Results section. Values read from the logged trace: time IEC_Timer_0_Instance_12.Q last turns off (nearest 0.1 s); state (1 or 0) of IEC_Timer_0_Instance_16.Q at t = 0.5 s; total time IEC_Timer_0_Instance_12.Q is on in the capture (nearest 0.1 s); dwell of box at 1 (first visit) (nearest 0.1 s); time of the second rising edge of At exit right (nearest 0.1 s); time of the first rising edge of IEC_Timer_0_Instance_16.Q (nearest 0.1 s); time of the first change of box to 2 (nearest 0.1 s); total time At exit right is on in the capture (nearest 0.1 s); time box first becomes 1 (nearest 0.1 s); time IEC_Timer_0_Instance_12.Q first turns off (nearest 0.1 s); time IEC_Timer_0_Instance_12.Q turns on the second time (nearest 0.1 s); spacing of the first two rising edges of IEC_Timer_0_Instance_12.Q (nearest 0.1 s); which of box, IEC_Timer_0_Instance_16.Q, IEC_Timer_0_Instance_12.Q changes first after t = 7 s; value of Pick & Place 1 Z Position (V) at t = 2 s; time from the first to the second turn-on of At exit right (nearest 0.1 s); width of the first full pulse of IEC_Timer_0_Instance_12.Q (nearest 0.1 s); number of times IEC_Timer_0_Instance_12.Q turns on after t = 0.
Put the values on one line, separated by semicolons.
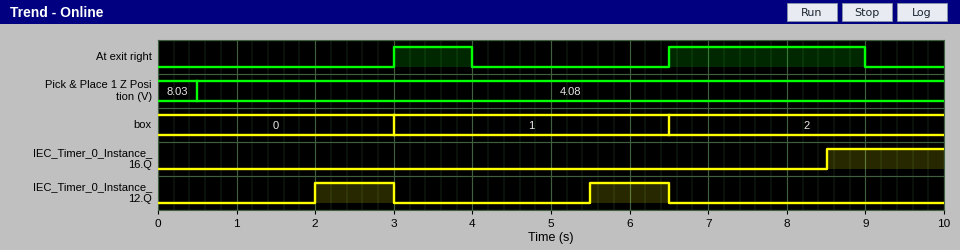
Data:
6.5 s; 0; 2.0 s; 3.5 s; 6.5 s; 8.5 s; 6.5 s; 3.5 s; 3.0 s; 3.0 s; 5.5 s; 3.5 s; IEC_Timer_0_Instance_16.Q; 4.08; 3.5 s; 1.0 s; 2
